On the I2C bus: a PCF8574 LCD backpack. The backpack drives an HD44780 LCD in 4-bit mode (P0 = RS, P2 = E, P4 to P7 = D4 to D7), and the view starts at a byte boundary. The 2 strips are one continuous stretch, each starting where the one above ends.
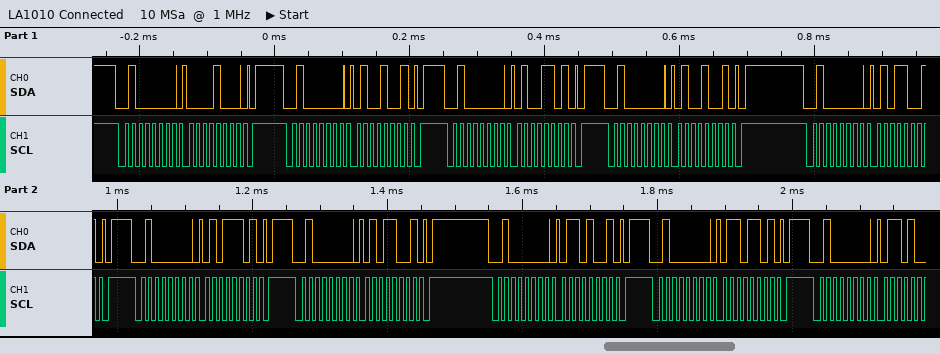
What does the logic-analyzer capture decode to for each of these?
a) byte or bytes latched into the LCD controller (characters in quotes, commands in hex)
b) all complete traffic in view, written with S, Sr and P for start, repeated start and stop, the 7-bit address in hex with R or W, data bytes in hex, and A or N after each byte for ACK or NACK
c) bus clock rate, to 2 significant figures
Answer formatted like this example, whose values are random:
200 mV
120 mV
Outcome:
'E'
S 20W A 08 A P S 20W A 49 A P S 20W A 4D A P S 20W A 49 A P S 20W A 59 A P S 20W A 5D A P S 20W A 59 A P S 20W A 69 A P S 20W A 6D A P S 20W A
100 kHz
